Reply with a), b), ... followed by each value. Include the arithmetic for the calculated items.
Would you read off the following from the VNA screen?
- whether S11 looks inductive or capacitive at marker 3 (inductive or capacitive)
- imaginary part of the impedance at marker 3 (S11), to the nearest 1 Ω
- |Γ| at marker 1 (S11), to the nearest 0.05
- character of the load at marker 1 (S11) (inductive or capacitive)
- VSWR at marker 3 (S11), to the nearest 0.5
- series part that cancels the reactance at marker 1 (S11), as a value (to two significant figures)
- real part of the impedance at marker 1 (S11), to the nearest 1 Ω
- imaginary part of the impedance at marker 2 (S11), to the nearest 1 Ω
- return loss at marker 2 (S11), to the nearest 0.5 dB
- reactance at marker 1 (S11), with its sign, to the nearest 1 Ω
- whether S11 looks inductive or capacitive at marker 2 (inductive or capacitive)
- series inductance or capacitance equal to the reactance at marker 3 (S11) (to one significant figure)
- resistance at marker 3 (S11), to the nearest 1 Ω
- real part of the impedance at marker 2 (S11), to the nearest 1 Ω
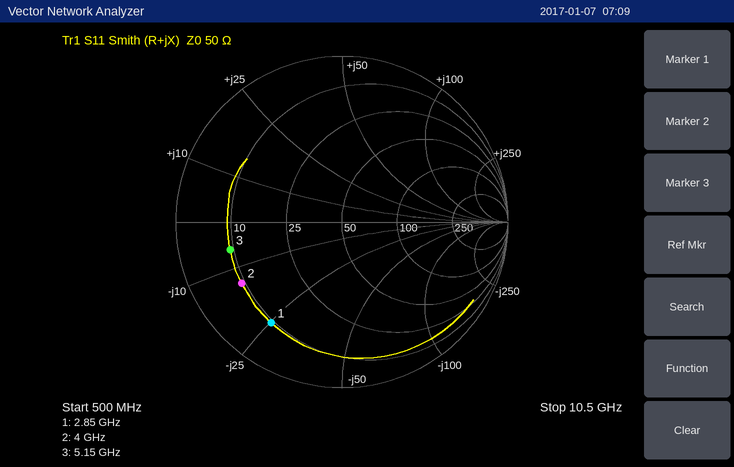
a) capacitive
b) -6 Ω
c) 0.75
d) capacitive
e) 5.5
f) L = 25 Ω/(2π × 2.85 GHz) ≈ 1.4 nH
g) 9 Ω
h) -14 Ω
i) 3.0 dB
j) -25 Ω
k) capacitive
l) C = 1/(2π × 5.15 GHz × 6 Ω) ≈ 5 pF
m) 9 Ω
n) 9 Ω
